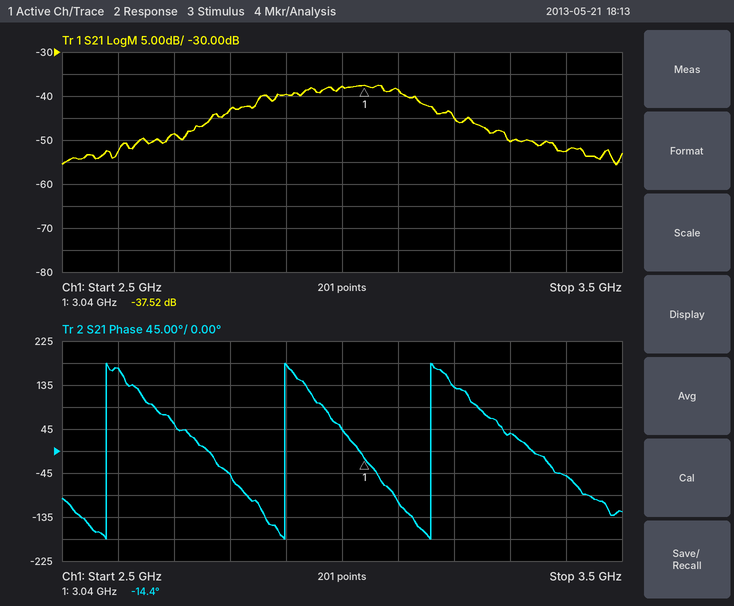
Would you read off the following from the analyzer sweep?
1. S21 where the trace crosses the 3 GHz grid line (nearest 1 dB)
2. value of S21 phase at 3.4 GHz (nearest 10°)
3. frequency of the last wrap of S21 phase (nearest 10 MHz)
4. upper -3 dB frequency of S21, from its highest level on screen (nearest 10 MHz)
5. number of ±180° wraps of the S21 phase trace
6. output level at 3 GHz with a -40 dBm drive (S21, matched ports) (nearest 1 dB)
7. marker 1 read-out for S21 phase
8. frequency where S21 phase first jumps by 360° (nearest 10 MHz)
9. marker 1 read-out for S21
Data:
-38 dB
-50°
3.16 GHz
3.13 GHz
3
-78 dBm
-14.4°
2.58 GHz
-37.52 dB
